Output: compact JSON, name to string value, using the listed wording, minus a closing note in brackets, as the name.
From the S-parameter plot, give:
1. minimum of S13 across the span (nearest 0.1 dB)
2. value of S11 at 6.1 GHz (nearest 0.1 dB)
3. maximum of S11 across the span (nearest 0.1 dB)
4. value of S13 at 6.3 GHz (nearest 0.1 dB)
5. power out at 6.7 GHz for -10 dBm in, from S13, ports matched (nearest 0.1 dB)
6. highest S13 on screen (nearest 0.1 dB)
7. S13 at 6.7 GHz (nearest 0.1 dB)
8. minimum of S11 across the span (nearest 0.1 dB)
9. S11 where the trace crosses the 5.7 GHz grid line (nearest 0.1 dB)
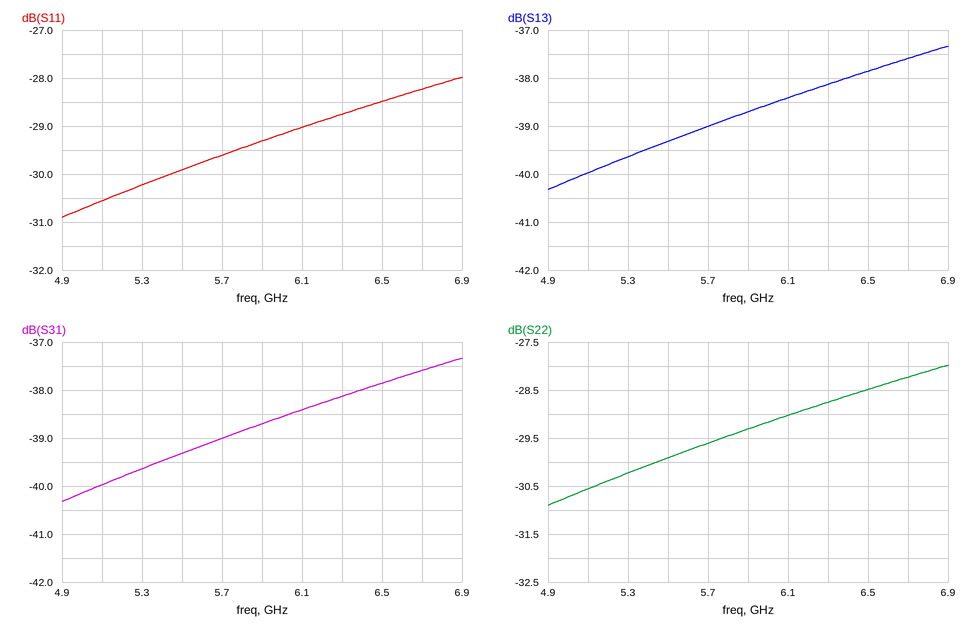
{"minimum of S13 across the span": "-40.3 dB", "value of S11 at 6.1 GHz": "-29.0 dB", "maximum of S11 across the span": "-28.0 dB", "value of S13 at 6.3 GHz": "-38.1 dB", "power out at 6.7 GHz for -10 dBm in, from S13, ports matched": "-47.6 dBm", "highest S13 on screen": "-37.3 dB", "S13 at 6.7 GHz": "-37.6 dB", "minimum of S11 across the span": "-30.9 dB", "S11 where the trace crosses the 5.7 GHz grid line": "-29.6 dB"}
